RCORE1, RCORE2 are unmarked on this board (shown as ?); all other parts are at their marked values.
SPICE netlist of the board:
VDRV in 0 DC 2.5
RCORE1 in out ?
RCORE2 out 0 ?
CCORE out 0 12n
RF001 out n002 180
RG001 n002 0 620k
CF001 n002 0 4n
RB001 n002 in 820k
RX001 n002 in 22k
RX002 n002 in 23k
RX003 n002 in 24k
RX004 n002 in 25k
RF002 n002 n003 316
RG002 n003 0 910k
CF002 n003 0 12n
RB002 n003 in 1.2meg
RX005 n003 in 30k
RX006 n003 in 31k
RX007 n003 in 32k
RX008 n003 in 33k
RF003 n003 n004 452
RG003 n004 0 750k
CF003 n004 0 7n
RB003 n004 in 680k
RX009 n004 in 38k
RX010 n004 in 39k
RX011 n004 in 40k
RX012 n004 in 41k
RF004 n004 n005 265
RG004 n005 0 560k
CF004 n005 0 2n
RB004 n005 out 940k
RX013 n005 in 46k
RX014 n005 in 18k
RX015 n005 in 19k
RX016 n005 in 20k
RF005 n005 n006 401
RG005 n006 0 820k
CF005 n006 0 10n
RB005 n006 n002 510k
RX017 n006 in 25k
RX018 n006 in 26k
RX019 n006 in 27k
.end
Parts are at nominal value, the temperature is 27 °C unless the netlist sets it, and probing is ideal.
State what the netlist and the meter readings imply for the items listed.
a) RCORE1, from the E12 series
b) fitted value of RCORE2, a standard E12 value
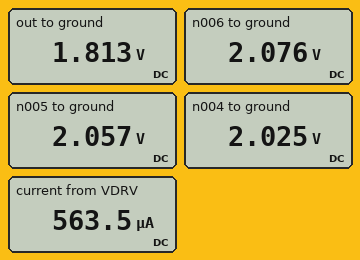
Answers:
3.3 kΩ
3.3 kΩ
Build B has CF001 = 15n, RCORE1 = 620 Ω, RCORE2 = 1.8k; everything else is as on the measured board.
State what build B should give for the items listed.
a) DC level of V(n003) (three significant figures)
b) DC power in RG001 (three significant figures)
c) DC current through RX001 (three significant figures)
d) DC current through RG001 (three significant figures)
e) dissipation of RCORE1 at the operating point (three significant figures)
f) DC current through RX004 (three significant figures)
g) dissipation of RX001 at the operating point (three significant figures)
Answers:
2.08 V
6.61 µW
21.6 µA
3.26 µA
440 µW
19.0 µA
10.3 µW
